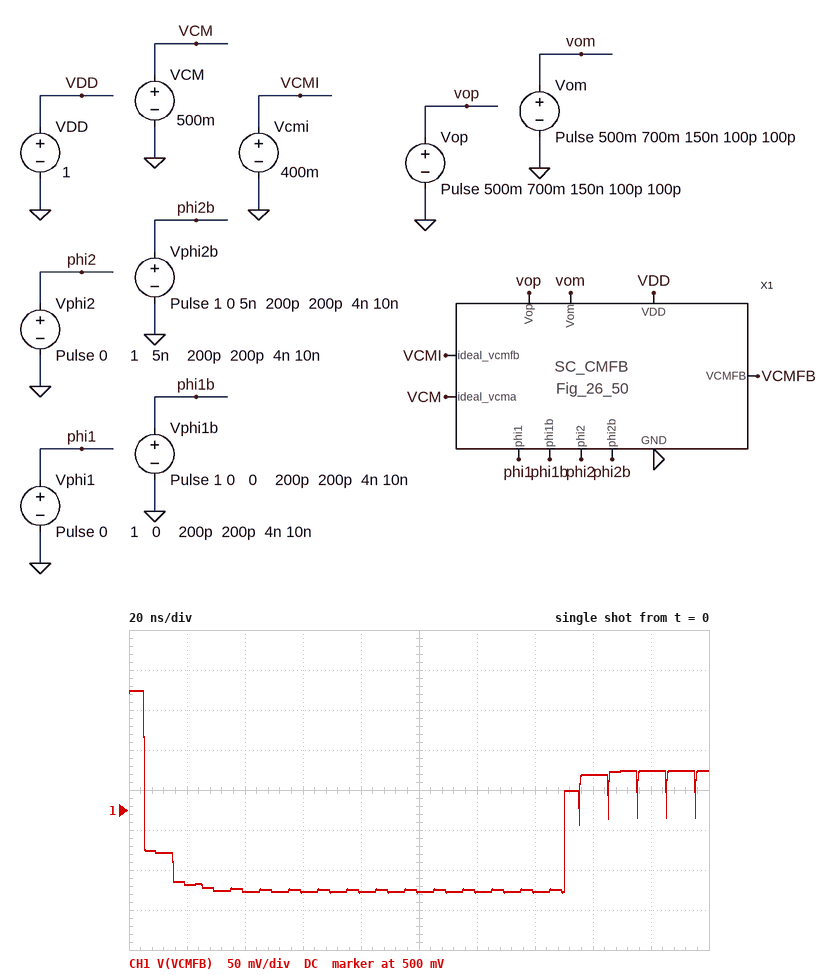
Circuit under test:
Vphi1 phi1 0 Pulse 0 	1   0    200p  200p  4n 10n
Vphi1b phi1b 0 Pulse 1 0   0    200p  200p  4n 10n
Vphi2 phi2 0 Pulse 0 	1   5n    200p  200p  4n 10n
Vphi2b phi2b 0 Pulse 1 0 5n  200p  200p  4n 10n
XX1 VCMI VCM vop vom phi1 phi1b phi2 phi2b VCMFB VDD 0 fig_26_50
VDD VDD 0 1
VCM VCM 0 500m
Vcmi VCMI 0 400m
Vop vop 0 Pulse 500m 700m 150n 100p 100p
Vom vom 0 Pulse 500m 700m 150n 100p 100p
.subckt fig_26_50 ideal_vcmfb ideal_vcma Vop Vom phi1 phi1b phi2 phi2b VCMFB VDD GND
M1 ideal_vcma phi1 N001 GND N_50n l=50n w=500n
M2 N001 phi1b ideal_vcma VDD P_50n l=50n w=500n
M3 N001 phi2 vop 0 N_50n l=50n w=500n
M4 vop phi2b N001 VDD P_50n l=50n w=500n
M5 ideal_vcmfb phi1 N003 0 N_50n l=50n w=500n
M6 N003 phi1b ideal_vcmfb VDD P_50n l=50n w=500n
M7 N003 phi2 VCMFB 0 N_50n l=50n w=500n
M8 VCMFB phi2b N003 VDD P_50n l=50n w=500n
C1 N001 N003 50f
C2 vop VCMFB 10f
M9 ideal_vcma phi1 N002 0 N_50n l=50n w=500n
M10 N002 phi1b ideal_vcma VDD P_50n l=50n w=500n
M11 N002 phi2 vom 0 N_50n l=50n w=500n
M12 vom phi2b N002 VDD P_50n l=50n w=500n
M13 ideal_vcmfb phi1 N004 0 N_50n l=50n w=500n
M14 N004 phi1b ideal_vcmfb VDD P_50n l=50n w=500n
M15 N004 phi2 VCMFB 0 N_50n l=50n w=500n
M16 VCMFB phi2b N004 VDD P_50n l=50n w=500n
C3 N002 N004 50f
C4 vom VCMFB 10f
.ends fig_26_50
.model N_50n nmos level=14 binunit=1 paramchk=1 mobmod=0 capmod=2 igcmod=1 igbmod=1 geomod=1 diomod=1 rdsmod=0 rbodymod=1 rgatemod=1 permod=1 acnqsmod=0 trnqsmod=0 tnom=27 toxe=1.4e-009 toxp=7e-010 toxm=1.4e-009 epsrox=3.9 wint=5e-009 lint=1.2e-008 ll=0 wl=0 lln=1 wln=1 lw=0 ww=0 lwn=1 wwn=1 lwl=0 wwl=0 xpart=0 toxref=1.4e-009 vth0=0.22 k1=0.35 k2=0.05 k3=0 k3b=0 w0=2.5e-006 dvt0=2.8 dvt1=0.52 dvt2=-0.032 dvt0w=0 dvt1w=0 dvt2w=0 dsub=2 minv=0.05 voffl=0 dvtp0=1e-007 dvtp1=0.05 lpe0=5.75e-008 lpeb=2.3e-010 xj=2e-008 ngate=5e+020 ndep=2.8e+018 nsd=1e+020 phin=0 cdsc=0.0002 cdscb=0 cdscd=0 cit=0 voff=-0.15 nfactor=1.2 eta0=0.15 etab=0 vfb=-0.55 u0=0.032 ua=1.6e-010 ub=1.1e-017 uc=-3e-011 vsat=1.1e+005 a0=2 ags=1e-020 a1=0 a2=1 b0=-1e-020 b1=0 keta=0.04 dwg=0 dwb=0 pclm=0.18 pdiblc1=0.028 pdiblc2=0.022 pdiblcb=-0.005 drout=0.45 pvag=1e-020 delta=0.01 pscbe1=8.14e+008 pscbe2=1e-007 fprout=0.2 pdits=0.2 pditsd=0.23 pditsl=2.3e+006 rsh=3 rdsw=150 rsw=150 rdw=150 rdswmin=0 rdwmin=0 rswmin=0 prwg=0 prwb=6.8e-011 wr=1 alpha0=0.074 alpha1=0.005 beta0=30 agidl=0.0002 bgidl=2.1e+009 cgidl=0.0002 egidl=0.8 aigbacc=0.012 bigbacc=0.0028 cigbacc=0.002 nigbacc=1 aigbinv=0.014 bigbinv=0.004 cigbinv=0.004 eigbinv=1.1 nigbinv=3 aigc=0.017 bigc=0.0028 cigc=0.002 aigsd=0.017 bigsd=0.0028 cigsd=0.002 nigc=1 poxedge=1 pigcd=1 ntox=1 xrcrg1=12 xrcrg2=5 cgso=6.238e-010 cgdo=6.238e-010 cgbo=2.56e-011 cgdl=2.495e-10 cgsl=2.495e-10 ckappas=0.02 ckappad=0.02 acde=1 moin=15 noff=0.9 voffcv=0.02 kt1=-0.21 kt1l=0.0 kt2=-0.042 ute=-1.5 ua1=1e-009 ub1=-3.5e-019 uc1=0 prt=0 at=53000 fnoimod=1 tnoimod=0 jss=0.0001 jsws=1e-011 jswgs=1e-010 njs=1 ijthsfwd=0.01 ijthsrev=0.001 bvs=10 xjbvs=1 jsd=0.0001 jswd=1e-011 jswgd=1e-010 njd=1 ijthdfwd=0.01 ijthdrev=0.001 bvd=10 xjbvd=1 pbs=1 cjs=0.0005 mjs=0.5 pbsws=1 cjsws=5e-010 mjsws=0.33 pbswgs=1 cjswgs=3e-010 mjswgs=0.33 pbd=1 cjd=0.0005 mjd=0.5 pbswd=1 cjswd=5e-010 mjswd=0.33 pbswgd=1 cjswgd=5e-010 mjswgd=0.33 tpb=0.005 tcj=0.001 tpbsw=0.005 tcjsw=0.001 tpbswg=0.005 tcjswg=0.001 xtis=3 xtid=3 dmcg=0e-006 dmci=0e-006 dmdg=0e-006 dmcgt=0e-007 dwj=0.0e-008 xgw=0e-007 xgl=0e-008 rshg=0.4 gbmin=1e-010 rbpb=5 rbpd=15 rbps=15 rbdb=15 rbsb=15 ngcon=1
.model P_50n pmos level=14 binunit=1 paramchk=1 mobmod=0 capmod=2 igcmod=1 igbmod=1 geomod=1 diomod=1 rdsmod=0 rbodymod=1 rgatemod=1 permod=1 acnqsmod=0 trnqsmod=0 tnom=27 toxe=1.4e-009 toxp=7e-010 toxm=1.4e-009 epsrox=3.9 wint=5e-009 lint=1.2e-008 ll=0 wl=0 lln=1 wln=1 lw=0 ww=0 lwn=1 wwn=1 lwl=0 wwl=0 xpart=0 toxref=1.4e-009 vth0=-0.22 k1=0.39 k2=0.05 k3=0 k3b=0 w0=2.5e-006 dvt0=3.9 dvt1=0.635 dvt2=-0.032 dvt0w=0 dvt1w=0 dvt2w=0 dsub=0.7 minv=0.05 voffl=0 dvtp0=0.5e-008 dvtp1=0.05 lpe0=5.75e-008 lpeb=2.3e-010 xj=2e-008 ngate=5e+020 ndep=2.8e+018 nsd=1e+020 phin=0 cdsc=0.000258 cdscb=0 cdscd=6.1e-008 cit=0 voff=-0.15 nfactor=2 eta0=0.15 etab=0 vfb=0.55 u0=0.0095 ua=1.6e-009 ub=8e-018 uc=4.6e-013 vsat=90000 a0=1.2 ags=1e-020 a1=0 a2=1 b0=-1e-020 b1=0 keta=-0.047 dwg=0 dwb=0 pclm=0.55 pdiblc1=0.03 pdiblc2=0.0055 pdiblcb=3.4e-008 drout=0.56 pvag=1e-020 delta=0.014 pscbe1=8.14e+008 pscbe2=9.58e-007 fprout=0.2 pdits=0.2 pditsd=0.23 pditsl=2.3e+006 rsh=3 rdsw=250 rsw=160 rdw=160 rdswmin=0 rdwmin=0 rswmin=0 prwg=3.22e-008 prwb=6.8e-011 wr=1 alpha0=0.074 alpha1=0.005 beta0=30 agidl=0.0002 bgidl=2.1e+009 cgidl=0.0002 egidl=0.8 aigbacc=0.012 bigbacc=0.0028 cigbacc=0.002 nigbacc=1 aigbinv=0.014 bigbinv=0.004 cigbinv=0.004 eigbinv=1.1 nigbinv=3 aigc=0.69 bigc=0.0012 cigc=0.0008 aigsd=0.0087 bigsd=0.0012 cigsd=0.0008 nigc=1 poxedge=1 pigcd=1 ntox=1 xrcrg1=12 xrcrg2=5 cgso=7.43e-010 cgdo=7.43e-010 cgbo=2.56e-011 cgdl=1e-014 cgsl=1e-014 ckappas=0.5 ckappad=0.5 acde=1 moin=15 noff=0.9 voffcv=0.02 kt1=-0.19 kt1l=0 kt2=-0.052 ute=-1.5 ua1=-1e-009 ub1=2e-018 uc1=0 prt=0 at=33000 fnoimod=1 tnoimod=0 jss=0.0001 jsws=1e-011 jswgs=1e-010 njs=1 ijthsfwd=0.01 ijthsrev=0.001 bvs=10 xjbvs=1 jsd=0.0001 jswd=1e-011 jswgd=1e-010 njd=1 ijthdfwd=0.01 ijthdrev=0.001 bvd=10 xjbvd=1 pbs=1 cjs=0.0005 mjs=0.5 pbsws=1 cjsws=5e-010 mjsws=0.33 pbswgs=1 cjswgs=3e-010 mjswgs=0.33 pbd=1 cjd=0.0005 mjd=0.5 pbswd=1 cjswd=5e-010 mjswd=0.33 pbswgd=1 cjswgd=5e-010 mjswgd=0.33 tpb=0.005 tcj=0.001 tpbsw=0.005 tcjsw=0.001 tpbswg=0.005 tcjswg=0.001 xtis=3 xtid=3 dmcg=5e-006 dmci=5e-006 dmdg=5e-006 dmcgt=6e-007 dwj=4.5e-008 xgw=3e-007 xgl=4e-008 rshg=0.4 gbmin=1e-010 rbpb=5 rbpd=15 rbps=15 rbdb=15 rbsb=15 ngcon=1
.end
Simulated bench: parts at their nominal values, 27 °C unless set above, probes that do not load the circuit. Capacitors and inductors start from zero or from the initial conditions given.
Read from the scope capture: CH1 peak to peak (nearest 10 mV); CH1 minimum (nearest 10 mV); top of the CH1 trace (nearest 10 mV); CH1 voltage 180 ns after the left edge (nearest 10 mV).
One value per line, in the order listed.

250 mV
400 mV
650 mV
550 mV
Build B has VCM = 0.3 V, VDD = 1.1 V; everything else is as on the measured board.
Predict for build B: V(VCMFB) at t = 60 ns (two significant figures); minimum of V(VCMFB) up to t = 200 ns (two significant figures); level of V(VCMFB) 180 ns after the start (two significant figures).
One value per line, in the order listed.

550 mV
510 mV
700 mV
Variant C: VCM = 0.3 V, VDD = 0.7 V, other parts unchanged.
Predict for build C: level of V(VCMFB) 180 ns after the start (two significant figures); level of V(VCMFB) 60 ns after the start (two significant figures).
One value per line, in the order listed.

690 mV
550 mV
